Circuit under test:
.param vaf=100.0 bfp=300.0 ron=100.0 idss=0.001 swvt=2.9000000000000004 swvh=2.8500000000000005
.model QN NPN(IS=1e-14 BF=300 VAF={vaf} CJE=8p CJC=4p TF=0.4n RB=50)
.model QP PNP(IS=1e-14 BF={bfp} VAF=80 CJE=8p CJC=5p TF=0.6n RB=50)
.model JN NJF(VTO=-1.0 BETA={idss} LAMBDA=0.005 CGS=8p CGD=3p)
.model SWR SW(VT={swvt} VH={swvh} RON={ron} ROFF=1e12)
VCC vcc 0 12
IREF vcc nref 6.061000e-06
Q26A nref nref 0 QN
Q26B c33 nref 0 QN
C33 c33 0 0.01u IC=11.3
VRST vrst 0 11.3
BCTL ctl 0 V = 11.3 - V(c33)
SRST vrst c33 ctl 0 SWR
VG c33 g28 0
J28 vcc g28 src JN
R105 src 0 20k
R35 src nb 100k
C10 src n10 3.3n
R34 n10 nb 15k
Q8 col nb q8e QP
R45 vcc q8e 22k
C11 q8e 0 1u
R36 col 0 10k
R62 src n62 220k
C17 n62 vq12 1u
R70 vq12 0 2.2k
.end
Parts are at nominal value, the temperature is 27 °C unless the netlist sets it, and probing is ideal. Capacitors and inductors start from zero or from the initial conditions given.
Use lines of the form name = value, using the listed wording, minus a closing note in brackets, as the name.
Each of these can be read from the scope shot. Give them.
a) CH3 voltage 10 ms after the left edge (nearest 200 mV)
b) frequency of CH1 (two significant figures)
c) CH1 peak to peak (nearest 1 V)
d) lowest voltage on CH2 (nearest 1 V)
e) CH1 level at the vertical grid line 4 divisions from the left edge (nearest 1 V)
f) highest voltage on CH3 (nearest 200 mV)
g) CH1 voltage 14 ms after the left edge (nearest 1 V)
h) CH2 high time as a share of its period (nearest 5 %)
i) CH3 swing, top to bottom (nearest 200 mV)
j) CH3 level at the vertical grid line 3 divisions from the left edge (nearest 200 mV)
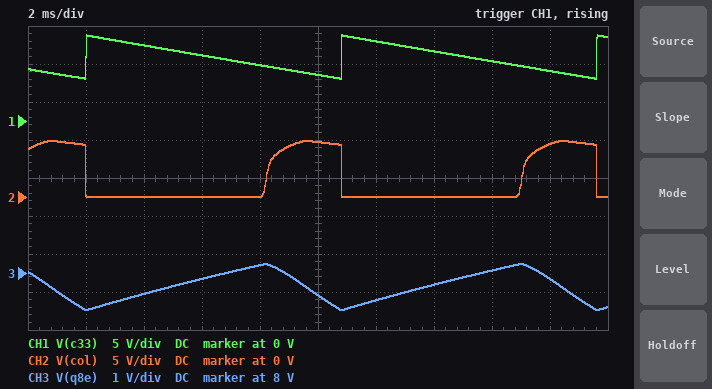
CH3 voltage 10 ms after the left edge = 7.4 V
frequency of CH1 = 110 Hz
CH1 peak to peak = 6 V
lowest voltage on CH2 = 0 V
CH1 level at the vertical grid line 4 divisions from the left edge = 7 V
highest voltage on CH3 = 8.2 V
CH1 voltage 14 ms after the left edge = 9 V
CH2 high time as a share of its period = 30 %
CH3 swing, top to bottom = 1.2 V
CH3 level at the vertical grid line 3 divisions from the left edge = 7.8 V
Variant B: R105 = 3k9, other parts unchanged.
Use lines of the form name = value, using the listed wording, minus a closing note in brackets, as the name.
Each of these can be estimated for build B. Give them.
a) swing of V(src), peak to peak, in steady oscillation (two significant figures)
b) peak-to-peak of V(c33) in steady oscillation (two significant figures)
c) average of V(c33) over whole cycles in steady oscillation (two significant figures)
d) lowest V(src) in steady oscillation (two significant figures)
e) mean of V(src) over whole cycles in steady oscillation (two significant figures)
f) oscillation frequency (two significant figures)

swing of V(src), peak to peak, in steady oscillation = 5.2 V
peak-to-peak of V(c33) in steady oscillation = 5.7 V
average of V(c33) over whole cycles in steady oscillation = 7.7 V
lowest V(src) in steady oscillation = 5.4 V
mean of V(src) over whole cycles in steady oscillation = 7.3 V
oscillation frequency = 150 Hz
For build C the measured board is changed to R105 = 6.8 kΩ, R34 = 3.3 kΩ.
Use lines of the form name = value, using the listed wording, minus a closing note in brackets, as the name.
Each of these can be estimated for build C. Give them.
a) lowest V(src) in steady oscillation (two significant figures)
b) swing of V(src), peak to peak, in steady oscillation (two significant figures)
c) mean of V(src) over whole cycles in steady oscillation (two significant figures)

lowest V(src) in steady oscillation = 5.7 V
swing of V(src), peak to peak, in steady oscillation = 5.3 V
mean of V(src) over whole cycles in steady oscillation = 8.3 V
